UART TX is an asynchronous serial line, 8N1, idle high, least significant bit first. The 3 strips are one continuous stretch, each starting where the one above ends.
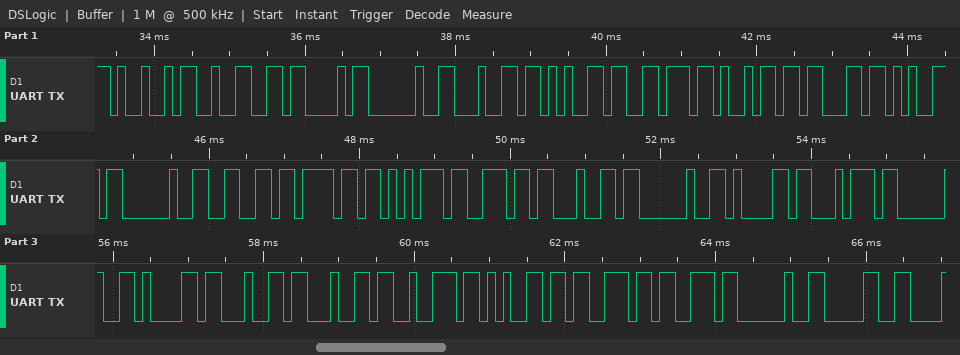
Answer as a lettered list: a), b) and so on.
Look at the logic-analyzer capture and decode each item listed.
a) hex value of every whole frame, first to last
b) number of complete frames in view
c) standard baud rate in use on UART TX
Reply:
a) 49 32 43 20 64 65 76 69 63 65 20 66 6F 75 6E 64 20 61 74 20 61 64 64 72 65 73 73 20 30
b) 29
c) 9600 baud
